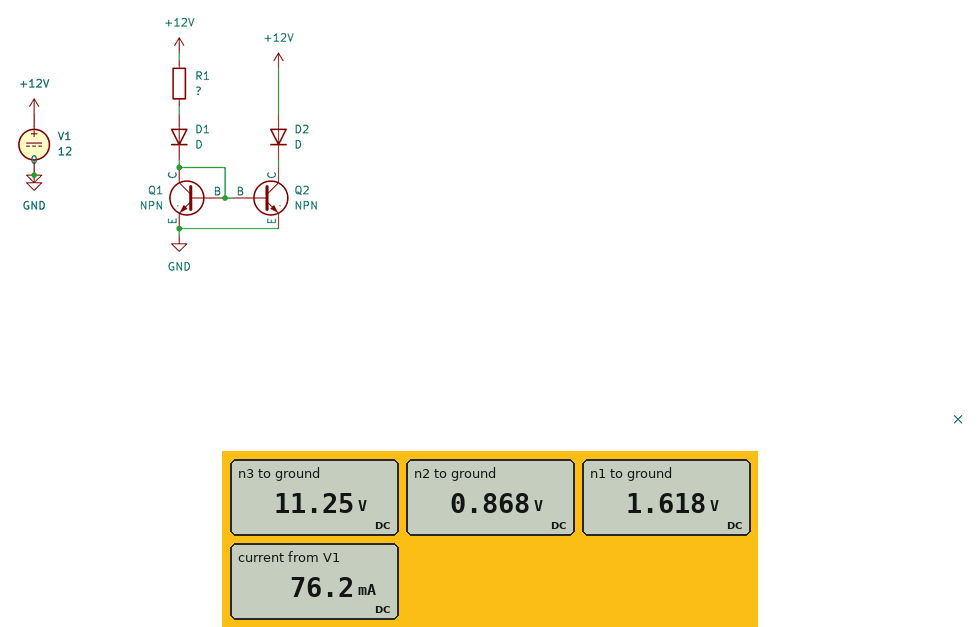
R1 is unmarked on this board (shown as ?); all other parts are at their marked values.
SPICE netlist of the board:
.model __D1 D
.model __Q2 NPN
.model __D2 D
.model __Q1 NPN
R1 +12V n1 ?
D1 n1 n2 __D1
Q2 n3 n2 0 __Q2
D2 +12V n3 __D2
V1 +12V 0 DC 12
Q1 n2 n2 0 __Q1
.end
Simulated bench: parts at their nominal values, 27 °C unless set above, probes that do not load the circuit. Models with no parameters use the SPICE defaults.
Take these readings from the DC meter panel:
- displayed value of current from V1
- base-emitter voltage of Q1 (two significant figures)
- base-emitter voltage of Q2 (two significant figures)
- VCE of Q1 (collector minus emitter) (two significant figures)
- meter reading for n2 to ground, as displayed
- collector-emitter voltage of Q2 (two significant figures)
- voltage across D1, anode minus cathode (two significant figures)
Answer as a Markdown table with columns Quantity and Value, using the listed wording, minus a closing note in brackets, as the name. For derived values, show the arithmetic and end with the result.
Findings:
| Quantity | Value |
|---|---|
| displayed value of current from V1 | 76.2 mA |
| base-emitter voltage of Q1 | 868 mV = 870 mV |
| base-emitter voltage of Q2 | 868 mV = 870 mV |
| VCE of Q1 (collector minus emitter) | 868 mV = 870 mV |
| meter reading for n2 to ground, as displayed | 0.868 V |
| collector-emitter voltage of Q2 | 11.25 V = 11 V |
| voltage across D1, anode minus cathode | 1.618 V - 868 mV = 750 mV |
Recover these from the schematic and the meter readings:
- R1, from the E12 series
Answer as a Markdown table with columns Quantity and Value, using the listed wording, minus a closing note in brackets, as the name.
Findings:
| Quantity | Value |
|---|---|
| R1, from the E12 series | 270 Ω |
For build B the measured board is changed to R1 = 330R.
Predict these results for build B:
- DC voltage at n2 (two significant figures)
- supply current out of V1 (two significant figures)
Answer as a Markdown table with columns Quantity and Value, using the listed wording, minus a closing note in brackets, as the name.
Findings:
| Quantity | Value |
|---|---|
| DC voltage at n2 | 860 mV |
| supply current out of V1 | 62 mA |
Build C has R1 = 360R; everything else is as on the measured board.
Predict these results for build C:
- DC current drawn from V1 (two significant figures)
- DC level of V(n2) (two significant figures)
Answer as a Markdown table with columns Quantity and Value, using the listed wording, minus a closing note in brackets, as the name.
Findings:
| Quantity | Value |
|---|---|
| DC current drawn from V1 | 57 mA |
| DC level of V(n2) | 860 mV |
